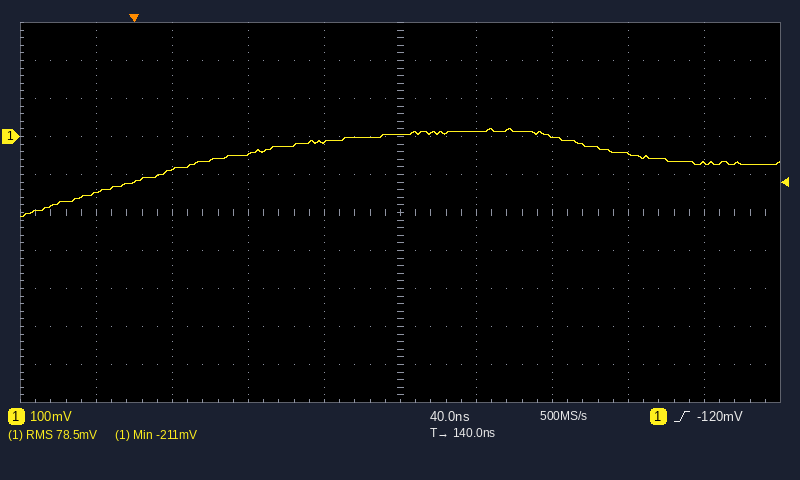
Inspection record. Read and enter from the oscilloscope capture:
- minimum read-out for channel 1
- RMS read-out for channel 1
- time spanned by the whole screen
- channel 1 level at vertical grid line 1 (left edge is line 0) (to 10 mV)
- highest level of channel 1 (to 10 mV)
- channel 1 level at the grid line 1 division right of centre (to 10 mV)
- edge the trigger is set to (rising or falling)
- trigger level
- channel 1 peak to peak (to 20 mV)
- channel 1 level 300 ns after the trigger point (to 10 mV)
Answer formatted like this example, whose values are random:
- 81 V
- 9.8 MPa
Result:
- -211 mV
- 78.5 mV
- 400 ns
- -150 mV
- 20 mV
- 10 mV
- rising
- -120 mV
- 240 mV
- -70 mV
